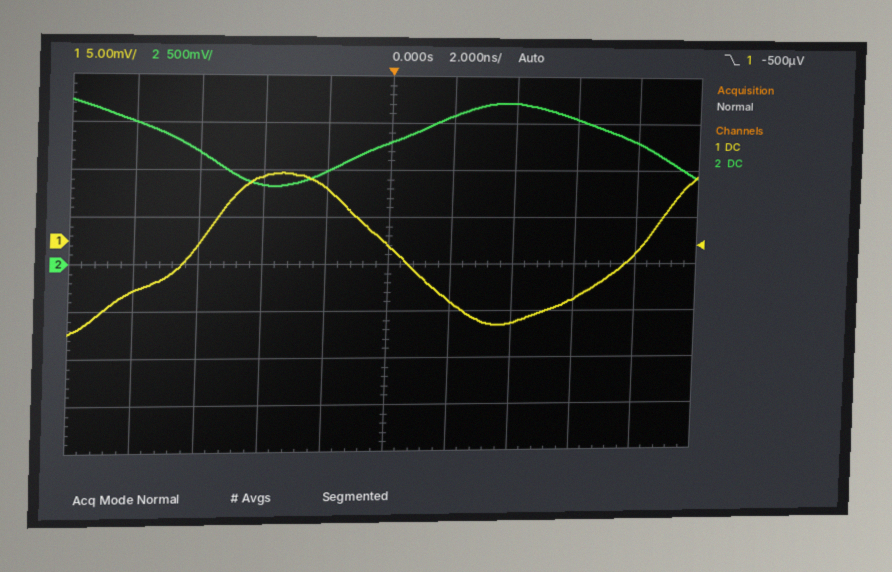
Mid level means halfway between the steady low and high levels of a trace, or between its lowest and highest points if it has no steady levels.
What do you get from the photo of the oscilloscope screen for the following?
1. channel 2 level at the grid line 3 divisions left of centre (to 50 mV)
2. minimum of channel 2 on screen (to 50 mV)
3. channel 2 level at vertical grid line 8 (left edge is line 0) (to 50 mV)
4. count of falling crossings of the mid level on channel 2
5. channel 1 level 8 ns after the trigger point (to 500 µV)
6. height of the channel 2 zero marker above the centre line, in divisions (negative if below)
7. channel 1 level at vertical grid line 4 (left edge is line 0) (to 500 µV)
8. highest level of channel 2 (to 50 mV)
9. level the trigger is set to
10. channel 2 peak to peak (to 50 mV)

1.20 V
850 mV
1.55 V
2
-1.5 mV
0.0 div
5.5 mV
1.75 V
-500 µV
900 mV
